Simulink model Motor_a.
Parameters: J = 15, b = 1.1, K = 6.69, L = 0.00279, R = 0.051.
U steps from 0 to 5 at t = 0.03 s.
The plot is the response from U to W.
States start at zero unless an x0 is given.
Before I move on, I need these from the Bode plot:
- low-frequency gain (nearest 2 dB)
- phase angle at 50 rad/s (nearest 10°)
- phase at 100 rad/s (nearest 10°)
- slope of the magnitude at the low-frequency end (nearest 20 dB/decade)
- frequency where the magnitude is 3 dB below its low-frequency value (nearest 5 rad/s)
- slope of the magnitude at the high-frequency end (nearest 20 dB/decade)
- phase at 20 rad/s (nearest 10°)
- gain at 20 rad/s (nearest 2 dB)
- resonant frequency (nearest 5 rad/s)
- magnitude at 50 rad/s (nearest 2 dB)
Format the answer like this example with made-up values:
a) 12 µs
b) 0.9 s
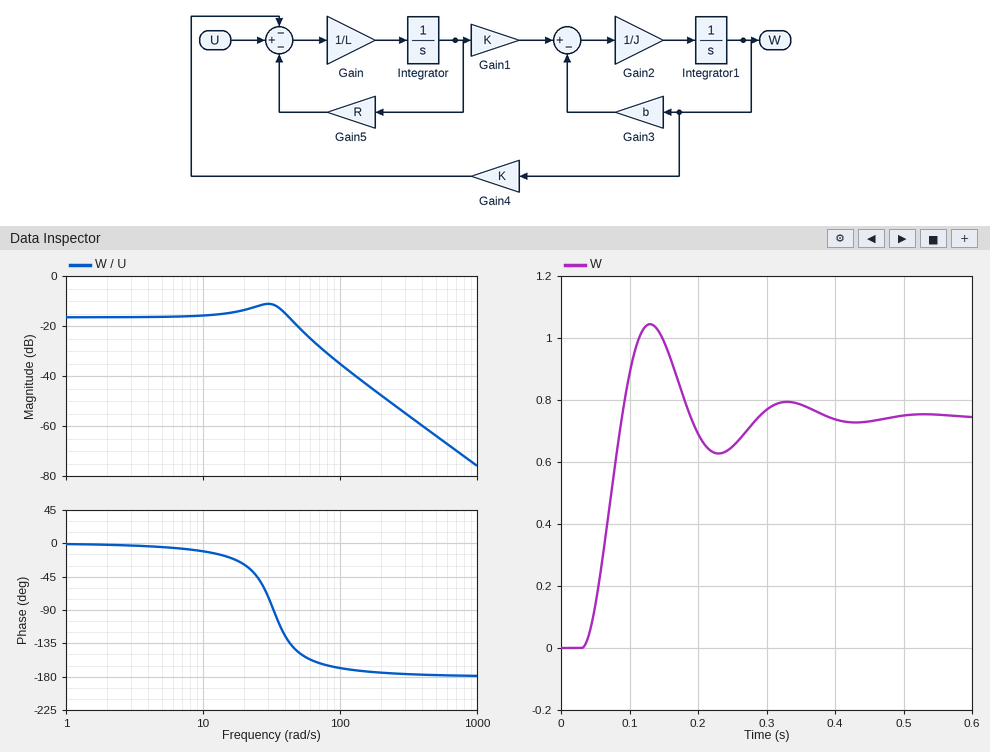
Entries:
a) -16 dB
b) -150°
c) -170°
d) 0 dB/decade
e) 50 rad/s
f) -40 dB/decade
g) -30°
h) -14 dB
i) 30 rad/s
j) -20 dB
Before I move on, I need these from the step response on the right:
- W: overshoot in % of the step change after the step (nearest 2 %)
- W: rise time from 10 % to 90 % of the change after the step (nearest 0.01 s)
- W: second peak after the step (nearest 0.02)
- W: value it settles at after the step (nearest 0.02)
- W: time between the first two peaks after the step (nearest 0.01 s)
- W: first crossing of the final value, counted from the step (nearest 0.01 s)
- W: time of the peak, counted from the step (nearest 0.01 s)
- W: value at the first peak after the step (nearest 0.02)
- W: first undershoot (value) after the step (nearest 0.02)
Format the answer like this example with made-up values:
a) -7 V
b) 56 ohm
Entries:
a) 40 %
b) 0.04 s
c) 0.80
d) 0.74
e) 0.20 s
f) 0.06 s
g) 0.10 s
h) 1.04
i) 0.62
